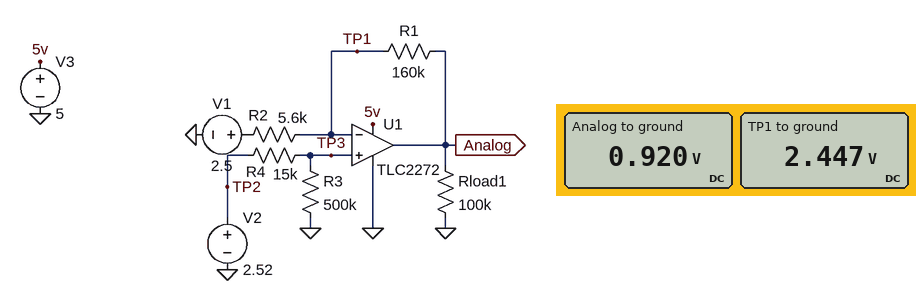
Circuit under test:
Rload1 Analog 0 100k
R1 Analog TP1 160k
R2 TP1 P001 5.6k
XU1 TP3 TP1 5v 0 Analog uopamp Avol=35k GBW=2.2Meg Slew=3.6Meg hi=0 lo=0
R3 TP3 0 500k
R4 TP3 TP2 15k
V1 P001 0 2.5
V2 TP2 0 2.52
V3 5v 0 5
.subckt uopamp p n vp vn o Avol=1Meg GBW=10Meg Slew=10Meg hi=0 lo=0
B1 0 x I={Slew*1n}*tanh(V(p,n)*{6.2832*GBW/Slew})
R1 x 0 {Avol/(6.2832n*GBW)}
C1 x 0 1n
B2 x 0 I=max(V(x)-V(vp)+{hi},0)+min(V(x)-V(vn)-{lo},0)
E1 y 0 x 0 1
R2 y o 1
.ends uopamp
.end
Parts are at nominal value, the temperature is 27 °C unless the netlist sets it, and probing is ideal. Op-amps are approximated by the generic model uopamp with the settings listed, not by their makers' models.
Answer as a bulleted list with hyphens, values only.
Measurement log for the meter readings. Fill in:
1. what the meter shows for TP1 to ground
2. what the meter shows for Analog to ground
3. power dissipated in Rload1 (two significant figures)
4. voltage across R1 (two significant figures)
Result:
- 2.447 V
- 0.920 V
- 8.5 µW
- 1.5 V
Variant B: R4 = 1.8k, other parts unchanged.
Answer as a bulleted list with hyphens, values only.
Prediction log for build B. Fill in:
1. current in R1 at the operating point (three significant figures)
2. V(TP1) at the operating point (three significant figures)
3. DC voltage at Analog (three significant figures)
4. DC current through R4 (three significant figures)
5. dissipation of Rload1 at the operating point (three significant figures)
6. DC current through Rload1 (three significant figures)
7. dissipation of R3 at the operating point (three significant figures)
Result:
- 1.94 µA
- 2.51 V
- 2.82 V
- 5.02 µA
- 79.6 µW
- 28.2 µA
- 12.6 µW
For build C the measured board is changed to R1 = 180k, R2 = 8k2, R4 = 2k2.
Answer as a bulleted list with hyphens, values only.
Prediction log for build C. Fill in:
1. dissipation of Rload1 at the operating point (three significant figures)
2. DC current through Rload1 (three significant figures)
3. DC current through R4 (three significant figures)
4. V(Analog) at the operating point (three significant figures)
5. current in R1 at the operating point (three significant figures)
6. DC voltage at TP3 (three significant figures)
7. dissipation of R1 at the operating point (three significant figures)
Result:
- 73.1 µW
- 27.0 µA
- 5.02 µA
- 2.70 V
- 1.08 µA
- 2.51 V
- 211 nW
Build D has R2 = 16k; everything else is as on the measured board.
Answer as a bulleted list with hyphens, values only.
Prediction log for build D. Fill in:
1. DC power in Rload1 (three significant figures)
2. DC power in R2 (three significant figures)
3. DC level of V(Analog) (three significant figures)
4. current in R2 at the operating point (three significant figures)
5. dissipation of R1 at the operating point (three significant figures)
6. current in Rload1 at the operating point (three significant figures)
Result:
- 36.6 µW
- 179 nW
- 1.91 V
- 3.34 µA
- 1.79 µW
- 19.1 µA
